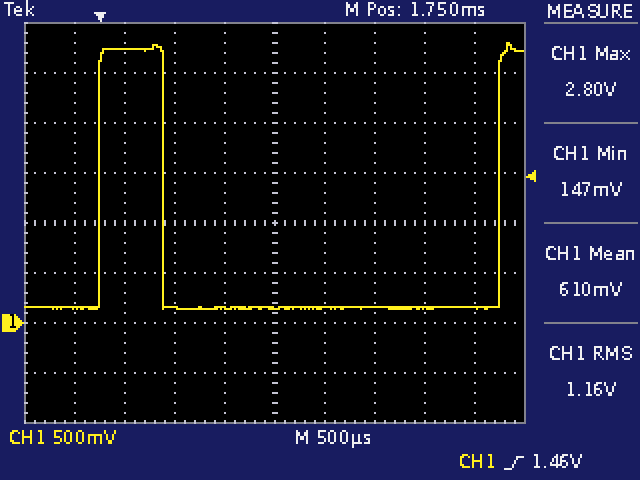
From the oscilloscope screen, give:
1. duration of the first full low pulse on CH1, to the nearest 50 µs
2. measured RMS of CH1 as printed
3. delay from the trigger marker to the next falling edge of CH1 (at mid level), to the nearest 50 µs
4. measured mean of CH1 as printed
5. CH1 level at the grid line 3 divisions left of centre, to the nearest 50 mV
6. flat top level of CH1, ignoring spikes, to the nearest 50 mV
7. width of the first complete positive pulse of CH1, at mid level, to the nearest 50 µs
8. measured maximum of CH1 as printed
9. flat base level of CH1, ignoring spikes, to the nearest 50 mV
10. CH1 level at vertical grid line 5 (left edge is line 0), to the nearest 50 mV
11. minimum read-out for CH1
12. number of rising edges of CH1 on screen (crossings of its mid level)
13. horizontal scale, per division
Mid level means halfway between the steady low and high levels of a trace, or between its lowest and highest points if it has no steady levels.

3.35 ms
1.16 V
650 µs
610 mV
2.75 V
2.75 V
650 µs
2.80 V
150 mV
150 mV
147 mV
2
500 µs
